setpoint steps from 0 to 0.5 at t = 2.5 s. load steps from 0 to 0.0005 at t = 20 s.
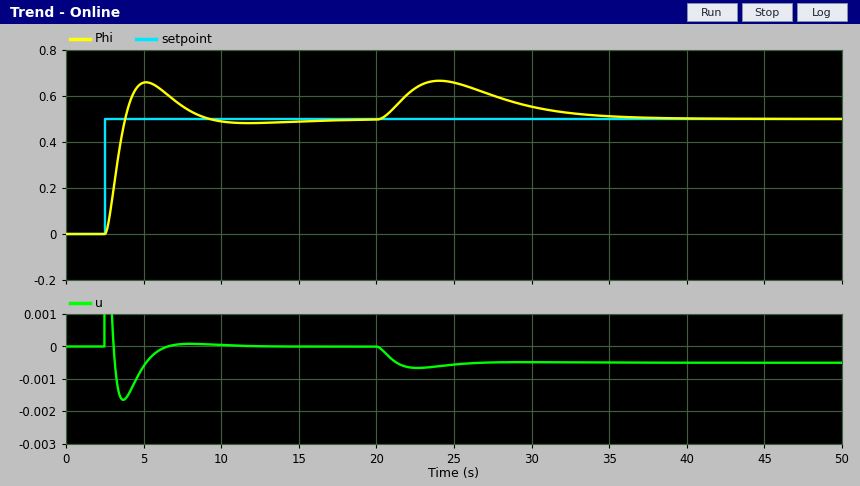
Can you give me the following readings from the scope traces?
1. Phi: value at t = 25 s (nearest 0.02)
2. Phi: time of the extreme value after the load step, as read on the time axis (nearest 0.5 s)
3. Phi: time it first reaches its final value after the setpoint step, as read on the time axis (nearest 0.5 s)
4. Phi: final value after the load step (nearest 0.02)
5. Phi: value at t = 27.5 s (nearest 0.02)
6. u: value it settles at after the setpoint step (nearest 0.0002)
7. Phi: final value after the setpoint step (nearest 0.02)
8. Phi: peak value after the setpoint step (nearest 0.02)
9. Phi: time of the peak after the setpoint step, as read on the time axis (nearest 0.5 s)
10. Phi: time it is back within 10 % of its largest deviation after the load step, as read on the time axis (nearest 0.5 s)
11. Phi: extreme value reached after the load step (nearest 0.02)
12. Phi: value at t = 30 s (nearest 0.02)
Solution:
0.66
24.0 s
4.0 s
0.50
0.60
0.0000
0.50
0.66
5.0 s
34.0 s
0.66
0.56
